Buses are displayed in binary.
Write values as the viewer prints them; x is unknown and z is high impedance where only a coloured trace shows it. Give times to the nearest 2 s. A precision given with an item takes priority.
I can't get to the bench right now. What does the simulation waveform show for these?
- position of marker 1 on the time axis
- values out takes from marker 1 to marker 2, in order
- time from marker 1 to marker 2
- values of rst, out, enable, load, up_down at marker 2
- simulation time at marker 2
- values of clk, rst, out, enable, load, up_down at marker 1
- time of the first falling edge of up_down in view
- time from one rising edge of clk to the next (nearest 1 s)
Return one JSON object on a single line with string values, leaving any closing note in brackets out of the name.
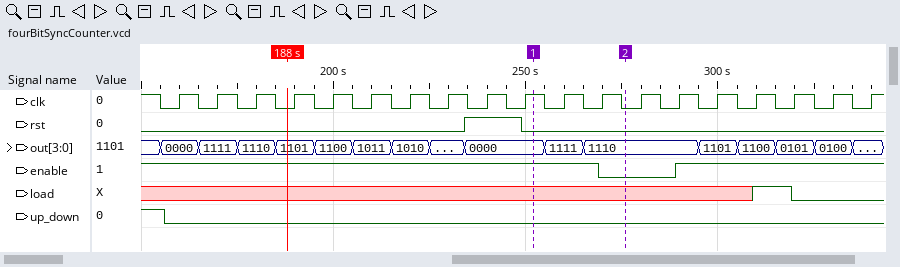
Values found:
{"position of marker 1 on the time axis": "252 s", "values out takes from marker 1 to marker 2, in order": "0000, 1111, 1110", "time from marker 1 to marker 2": "24 s", "values of rst, out, enable, load, up_down at marker 2": "rst=0, out=1110, enable=0, load=x, up_down=0", "simulation time at marker 2": "276 s", "values of clk, rst, out, enable, load, up_down at marker 1": "clk=1, rst=0, out=0000, enable=1, load=x, up_down=0", "time of the first falling edge of up_down in view": "156 s", "time from one rising edge of clk to the next": "10 s"}
